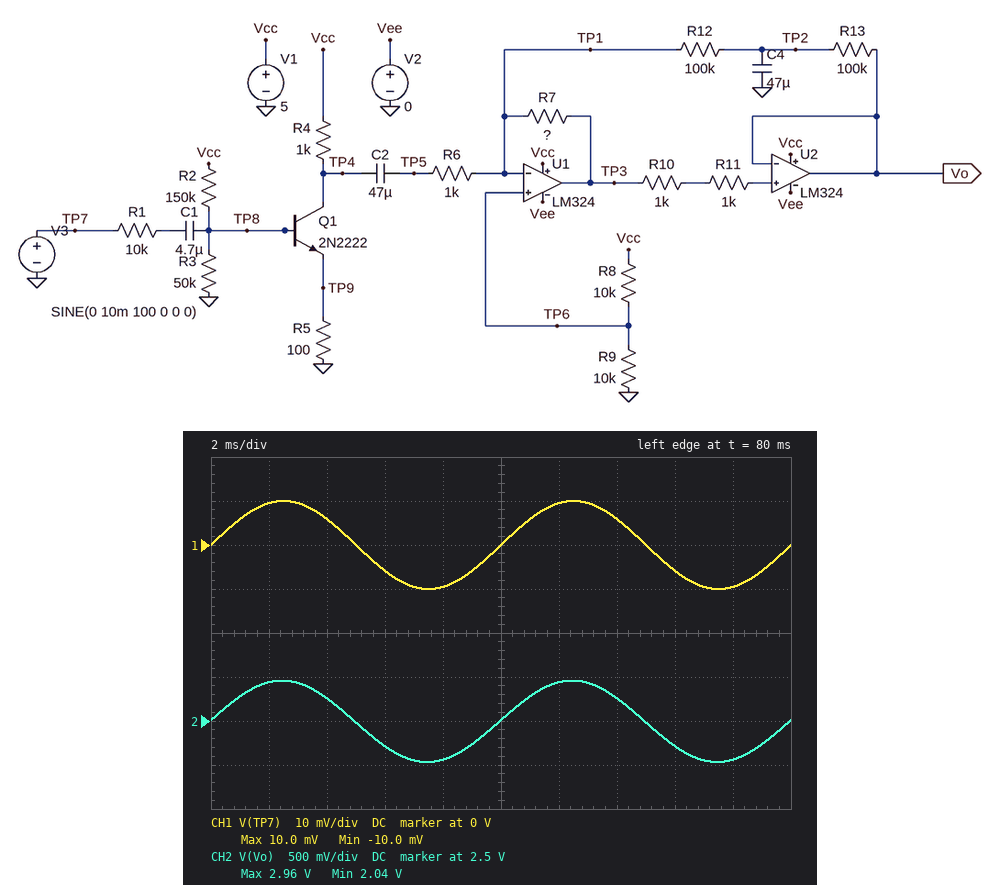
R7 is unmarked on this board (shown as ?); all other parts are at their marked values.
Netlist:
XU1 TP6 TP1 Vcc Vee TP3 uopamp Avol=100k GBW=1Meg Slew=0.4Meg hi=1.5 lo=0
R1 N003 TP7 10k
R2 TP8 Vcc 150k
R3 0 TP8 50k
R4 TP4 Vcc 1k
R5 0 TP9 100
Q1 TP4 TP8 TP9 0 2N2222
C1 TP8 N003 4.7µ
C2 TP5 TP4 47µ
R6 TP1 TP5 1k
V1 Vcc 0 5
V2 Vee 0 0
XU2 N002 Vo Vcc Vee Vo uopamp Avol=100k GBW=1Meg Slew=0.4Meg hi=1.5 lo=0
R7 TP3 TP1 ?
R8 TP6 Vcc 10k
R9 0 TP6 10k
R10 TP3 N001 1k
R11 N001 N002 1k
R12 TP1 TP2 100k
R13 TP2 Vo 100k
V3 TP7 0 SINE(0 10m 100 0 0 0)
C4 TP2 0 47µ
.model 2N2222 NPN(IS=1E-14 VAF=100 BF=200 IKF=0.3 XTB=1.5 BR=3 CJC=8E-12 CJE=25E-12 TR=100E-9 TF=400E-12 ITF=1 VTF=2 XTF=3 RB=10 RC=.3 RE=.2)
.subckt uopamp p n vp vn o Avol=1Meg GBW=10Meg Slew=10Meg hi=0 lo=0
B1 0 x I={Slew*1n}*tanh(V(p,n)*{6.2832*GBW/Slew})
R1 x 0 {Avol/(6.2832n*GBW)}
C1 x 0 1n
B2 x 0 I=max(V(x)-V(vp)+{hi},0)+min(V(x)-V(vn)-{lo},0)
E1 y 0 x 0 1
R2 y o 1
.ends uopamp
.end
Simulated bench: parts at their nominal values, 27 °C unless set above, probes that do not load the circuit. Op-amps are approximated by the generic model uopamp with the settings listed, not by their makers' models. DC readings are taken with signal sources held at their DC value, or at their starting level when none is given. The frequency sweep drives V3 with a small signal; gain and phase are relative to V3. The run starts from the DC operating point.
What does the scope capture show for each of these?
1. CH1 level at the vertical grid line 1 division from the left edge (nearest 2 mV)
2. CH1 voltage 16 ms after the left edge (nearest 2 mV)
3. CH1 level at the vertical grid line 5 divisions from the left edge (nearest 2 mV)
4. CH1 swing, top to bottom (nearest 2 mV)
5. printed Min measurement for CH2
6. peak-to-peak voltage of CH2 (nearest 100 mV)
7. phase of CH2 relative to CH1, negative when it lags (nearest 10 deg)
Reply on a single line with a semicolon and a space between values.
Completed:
10 mV; -6 mV; 0 V; 20 mV; 2.04 V; 900 mV; 0 deg
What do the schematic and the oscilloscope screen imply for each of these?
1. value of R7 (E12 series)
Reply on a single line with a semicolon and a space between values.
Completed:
18 kΩ
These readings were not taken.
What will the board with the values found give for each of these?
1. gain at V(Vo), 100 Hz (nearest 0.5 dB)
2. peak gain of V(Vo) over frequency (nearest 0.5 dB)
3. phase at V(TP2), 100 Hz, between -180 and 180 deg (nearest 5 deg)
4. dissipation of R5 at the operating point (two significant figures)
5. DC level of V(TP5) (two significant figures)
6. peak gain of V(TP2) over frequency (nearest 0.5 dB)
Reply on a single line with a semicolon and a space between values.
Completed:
33.5 dB; 33.5 dB; -90 deg; 410 µW; 2.5 V; -6.0 dB
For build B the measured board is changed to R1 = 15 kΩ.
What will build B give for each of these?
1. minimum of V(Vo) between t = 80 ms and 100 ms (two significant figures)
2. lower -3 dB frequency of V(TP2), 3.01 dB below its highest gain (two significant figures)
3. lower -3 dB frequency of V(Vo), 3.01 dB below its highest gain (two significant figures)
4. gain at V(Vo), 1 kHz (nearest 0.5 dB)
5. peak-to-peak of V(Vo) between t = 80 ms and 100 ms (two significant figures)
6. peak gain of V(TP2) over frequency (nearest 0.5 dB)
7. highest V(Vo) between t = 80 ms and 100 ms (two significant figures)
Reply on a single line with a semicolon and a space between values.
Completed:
2.1 V; 580 mHz; 2.2 Hz; 31.5 dB; 770 mV; -7.0 dB; 2.9 V
